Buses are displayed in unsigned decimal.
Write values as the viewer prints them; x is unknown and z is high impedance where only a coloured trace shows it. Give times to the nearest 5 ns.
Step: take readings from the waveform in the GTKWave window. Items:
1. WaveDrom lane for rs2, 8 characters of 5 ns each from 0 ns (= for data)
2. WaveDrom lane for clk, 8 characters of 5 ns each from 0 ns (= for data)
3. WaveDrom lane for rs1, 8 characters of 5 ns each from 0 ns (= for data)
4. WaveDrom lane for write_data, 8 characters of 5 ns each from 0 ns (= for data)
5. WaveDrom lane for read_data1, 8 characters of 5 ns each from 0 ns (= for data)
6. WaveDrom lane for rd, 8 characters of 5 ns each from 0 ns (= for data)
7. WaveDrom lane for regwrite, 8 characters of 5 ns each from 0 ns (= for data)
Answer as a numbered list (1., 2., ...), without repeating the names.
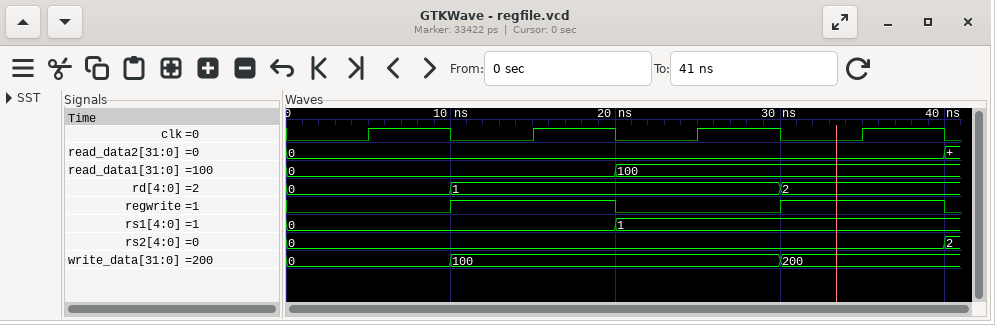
1. {name: 'rs2', wave: '=.......', data: '0'}
2. {name: 'clk', wave: '01010101'}
3. {name: 'rs1', wave: '=...=...', data: '0 1'}
4. {name: 'write_data', wave: '=.=...=.', data: '0 100 200'}
5. {name: 'read_data1', wave: '=...=...', data: '0 100'}
6. {name: 'rd', wave: '=.=...=.', data: '0 1 2'}
7. {name: 'regwrite', wave: '0.1.0.1.'}
